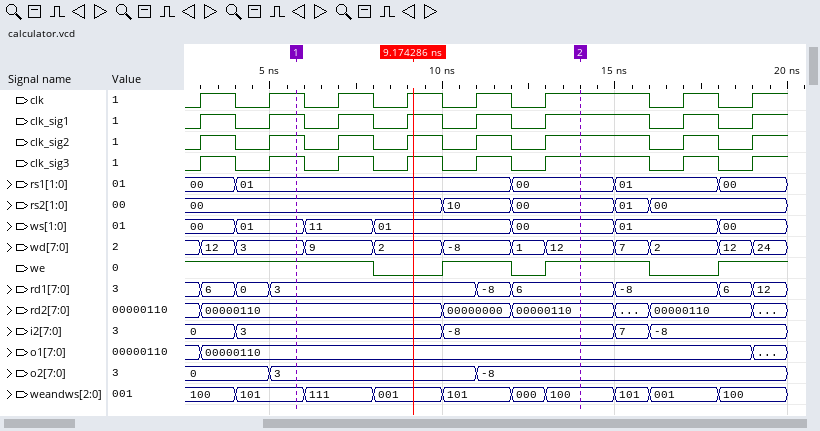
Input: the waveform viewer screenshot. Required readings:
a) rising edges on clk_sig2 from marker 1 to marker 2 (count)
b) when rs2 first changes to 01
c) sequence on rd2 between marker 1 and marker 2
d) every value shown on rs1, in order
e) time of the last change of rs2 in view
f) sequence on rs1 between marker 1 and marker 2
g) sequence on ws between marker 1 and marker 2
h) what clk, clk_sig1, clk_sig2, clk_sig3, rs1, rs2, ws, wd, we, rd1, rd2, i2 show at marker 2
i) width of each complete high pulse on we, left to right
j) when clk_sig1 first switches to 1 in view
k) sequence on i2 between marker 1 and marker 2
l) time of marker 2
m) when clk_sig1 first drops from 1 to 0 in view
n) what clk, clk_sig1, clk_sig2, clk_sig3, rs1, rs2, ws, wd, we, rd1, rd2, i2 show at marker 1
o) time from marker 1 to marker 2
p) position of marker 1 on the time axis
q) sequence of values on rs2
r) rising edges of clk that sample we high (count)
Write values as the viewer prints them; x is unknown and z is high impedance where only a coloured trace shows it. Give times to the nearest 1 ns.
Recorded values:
4
15 ns
00000110, 00000000, 00000110
00, 01, 00, 01, 00
16 ns
01, 00
01, 11, 01, 00
clk=1, clk_sig1=1, clk_sig2=1, clk_sig3=1, rs1=00, rs2=00, ws=00, wd=12, we=1, rd1=6, rd2=00000110, i2=-8
2 ns, 3 ns
3 ns
3, -8
14 ns
4 ns
clk=1, clk_sig1=1, clk_sig2=1, clk_sig3=1, rs1=01, rs2=00, ws=01, wd=3, we=1, rd1=3, rd2=00000110, i2=3
8 ns
6 ns
00, 10, 00, 01, 00
5
